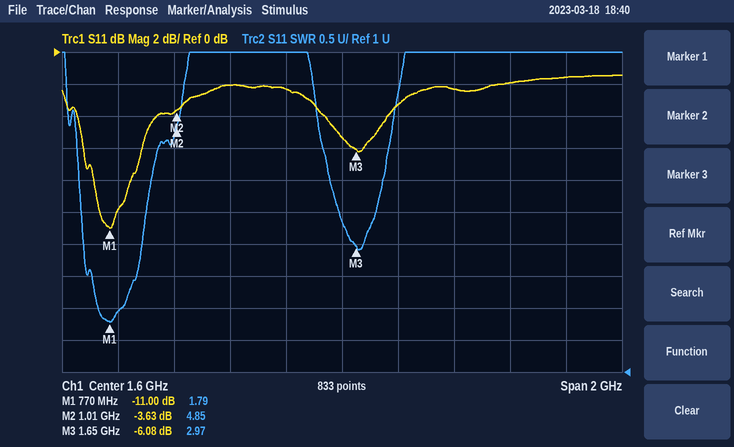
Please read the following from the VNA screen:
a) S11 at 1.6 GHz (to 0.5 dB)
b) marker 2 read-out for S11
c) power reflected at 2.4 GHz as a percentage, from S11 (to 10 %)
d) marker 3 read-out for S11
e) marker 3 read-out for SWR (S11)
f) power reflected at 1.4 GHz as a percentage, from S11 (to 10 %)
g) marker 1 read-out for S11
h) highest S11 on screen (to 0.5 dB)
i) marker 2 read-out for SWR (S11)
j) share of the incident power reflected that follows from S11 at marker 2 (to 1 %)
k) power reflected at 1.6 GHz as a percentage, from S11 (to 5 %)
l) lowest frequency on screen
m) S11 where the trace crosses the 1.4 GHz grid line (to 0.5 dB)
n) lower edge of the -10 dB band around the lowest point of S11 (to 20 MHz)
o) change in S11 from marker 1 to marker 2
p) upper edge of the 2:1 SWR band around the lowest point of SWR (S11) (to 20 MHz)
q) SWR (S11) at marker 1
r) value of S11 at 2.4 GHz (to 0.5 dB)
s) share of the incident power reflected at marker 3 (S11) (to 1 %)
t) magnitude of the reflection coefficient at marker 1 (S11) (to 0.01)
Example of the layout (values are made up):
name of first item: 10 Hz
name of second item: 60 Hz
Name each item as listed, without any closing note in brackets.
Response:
S11 at 1.6 GHz: -5.5 dB
marker 2 read-out for S11: -3.63 dB
power reflected at 2.4 GHz as a percentage, from S11: 70 %
marker 3 read-out for S11: -6.08 dB
marker 3 read-out for SWR: 2.97
power reflected at 1.4 GHz as a percentage, from S11: 60 %
marker 1 read-out for S11: -11.00 dB
highest S11 on screen: -1.5 dB
marker 2 read-out for SWR: 4.85
share of the incident power reflected that follows from S11 at marker 2: 43 %
power reflected at 1.6 GHz as a percentage, from S11: 30 %
lowest frequency on screen: 600 MHz
S11 where the trace crosses the 1.4 GHz grid line: -2.5 dB
lower edge of the -10 dB band around the lowest point of S11: 740 MHz
change in S11 from marker 1 to marker 2: 7.37 dB
upper edge of the 2:1 SWR band around the lowest point of SWR (S11): 820 MHz
SWR (S11) at marker 1: 1.79
value of S11 at 2.4 GHz: -1.5 dB
share of the incident power reflected at marker 3 (S11): 25 %
magnitude of the reflection coefficient at marker 1 (S11): 0.28
